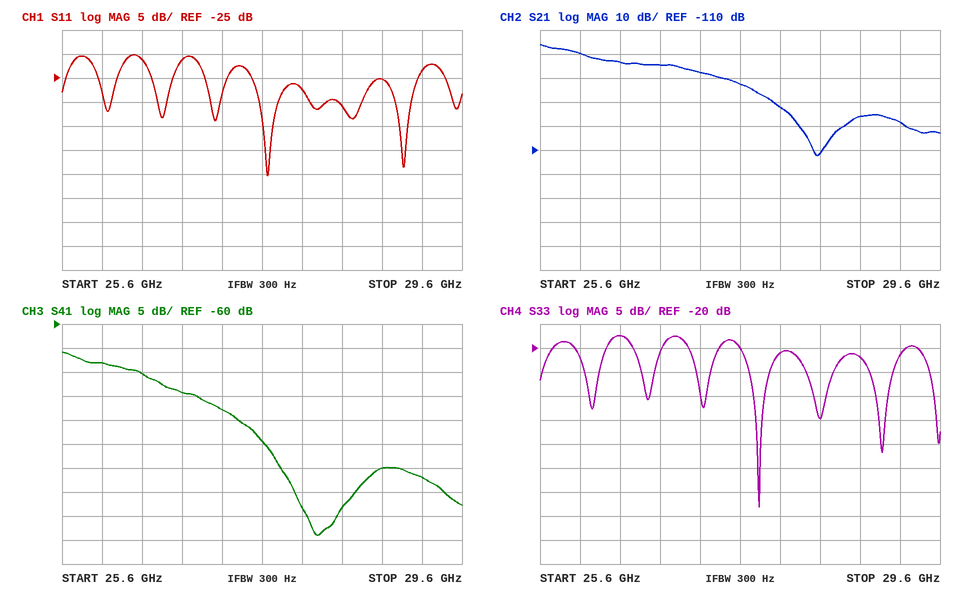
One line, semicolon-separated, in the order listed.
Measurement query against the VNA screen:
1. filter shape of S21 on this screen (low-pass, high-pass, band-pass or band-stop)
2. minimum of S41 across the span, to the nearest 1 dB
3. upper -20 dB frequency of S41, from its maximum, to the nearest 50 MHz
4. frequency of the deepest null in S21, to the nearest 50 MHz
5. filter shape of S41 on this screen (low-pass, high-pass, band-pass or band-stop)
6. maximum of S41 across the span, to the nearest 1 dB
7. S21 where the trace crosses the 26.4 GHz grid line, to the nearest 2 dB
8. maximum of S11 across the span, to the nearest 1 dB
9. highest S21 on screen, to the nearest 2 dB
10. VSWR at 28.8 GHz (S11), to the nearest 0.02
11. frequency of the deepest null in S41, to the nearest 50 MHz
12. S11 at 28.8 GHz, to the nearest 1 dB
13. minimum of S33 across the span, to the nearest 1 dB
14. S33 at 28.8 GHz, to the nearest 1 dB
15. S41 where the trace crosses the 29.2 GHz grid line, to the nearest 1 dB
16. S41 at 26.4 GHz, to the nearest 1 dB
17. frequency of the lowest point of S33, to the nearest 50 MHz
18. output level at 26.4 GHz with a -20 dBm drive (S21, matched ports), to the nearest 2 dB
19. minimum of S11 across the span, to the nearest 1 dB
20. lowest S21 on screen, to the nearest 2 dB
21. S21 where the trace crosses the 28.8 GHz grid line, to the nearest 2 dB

low-pass; -104 dB; 27.65 GHz; 28.35 GHz; low-pass; -66 dB; -74 dB; -20 dB; -66 dB; 1.12; 28.15 GHz; -25 dB; -53 dB; -22 dB; -92 dB; -70 dB; 27.80 GHz; -94 dBm; -45 dB; -112 dB; -96 dB
